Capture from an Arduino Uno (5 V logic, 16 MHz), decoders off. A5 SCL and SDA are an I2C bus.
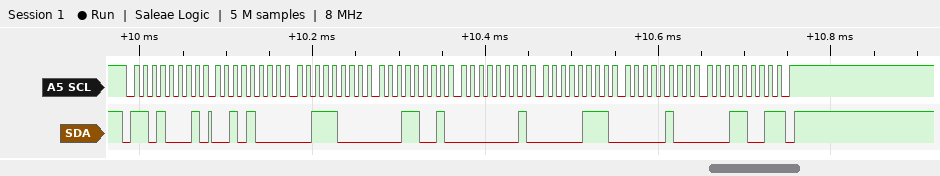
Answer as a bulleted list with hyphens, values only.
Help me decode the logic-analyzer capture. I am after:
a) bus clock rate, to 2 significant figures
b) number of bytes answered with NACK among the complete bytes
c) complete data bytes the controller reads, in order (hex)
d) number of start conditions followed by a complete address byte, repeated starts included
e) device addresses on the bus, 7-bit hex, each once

- 100 kHz
- 1
- 28 38 19 01 07 04 19
- 1
- 0x68
